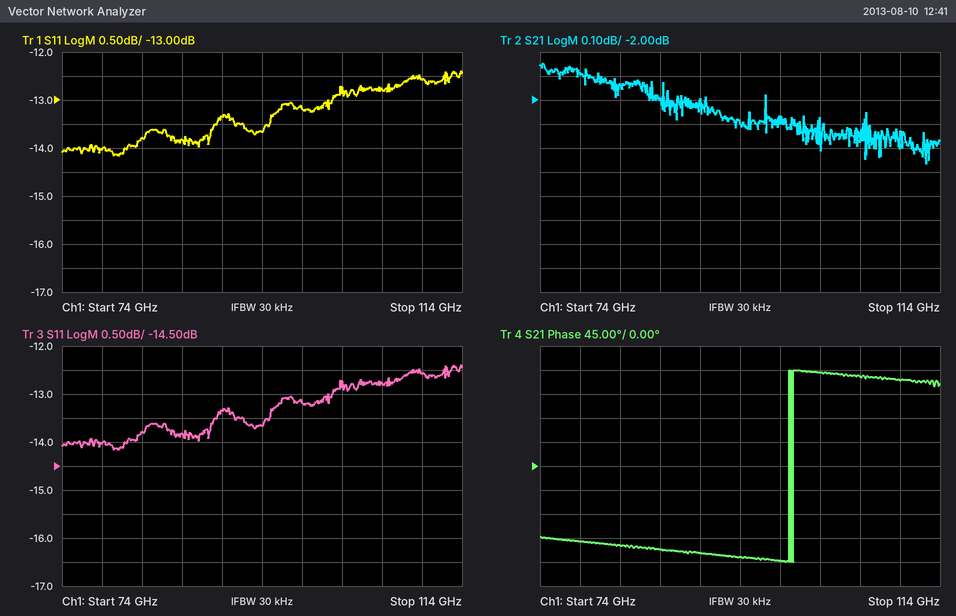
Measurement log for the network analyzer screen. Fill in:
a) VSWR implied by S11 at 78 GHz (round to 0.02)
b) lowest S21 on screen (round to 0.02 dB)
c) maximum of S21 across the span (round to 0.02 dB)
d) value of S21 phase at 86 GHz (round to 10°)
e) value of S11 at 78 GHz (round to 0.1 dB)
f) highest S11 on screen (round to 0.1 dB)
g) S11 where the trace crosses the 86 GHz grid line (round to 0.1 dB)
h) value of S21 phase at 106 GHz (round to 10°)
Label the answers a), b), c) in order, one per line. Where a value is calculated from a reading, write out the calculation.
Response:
a) |Γ| = 10^(-14/20) = 0.1995; VSWR = (1 + 0.1995)/(1 − 0.1995) ≈ 1.50
b) -2.26 dB
c) -1.84 dB
d) -160°
e) -14.0 dB
f) -12.4 dB
g) -13.8 dB
h) 170°
